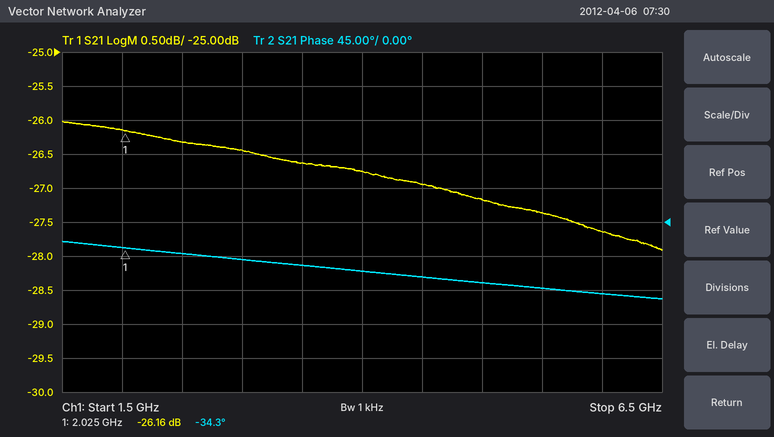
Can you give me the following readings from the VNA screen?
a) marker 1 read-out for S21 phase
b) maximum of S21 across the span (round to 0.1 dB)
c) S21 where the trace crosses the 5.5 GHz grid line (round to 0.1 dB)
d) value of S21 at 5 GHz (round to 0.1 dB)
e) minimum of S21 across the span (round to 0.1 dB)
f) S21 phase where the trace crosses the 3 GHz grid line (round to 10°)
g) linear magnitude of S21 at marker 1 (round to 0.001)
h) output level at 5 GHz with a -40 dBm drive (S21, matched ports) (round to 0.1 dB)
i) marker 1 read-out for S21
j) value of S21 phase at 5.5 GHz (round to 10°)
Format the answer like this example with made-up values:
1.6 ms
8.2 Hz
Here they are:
-34.3°
-26.0 dB
-27.4 dB
-27.2 dB
-27.9 dB
-50°
0.049
-67.2 dBm
-26.16 dB
-90°
